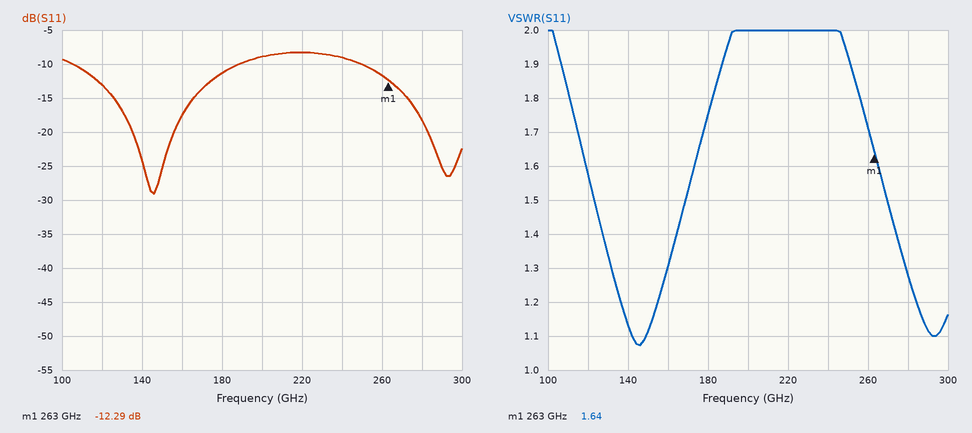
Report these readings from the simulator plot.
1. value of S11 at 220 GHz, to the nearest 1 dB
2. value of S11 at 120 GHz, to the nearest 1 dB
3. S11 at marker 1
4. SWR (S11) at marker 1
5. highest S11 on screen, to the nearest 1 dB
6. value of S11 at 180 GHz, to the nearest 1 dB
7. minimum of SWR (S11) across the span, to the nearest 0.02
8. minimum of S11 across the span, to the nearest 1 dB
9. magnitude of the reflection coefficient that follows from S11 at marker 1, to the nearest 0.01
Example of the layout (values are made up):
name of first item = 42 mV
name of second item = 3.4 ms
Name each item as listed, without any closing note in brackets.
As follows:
value of S11 at 220 GHz, to the nearest 1 dB = -8 dB
value of S11 at 120 GHz, to the nearest 1 dB = -13 dB
S11 at marker 1 = -12.29 dB
SWR (S11) at marker 1 = 1.64
highest S11 on screen, to the nearest 1 dB = -8 dB
value of S11 at 180 GHz, to the nearest 1 dB = -11 dB
minimum of SWR (S11) across the span, to the nearest 0.02 = 1.08
minimum of S11 across the span, to the nearest 1 dB = -29 dB
magnitude of the reflection coefficient that follows from S11 at marker 1, to the nearest 0.01 = 0.24
